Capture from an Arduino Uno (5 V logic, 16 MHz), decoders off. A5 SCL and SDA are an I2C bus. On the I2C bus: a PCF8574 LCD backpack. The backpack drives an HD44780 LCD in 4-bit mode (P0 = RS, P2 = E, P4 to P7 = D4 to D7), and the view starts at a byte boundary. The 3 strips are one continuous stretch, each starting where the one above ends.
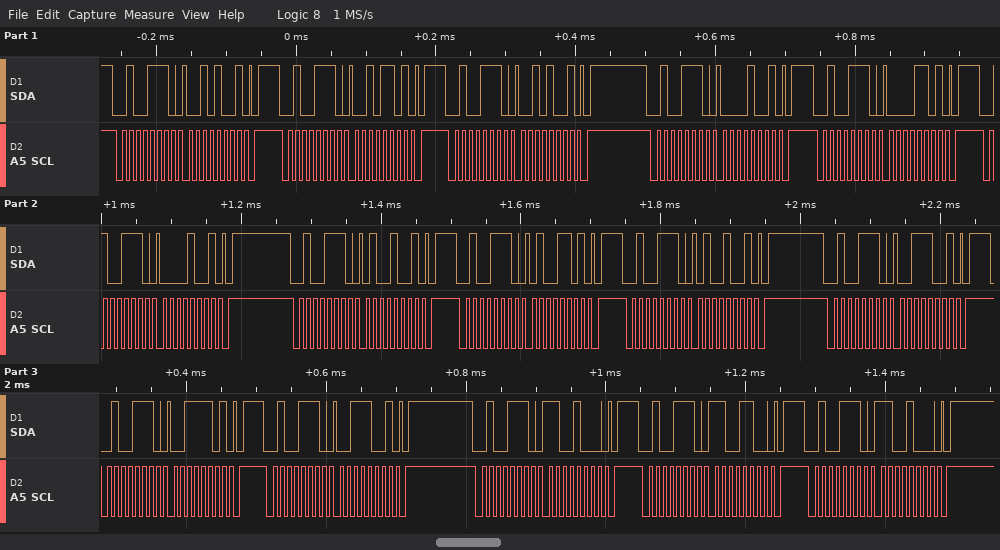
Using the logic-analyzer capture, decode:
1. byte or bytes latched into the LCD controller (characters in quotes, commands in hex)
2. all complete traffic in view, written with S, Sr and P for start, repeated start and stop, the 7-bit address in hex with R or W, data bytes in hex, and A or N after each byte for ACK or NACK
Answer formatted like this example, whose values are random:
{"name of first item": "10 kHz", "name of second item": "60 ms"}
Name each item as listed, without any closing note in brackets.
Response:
{"byte or bytes latched into the LCD controller": "' ' 'C'", "all complete traffic in view, written with S, Sr and P for start, repeated start and stop, the 7-bit address in hex with R or W, data bytes in hex, and A or N after each byte for ACK or NACK": "S 27W A 29 A P S 27W A 2D A P S 27W A 29 A P S 27W A 09 A P S 27W A 0D A P S 27W A 09 A P S 27W A 49 A P S 27W A 4D A P S 27W A 49 A P S 27W A 39 A P S 27W A 3D A P S 27W A 39 A P S 27W A C8 A P S 27W A CC A P S 27W A C8 A P"}
